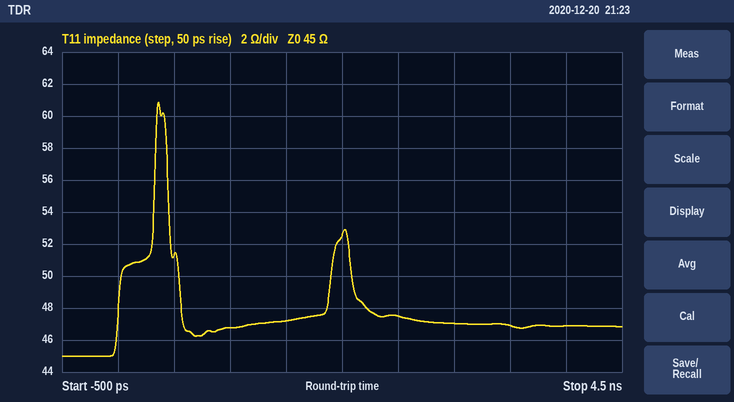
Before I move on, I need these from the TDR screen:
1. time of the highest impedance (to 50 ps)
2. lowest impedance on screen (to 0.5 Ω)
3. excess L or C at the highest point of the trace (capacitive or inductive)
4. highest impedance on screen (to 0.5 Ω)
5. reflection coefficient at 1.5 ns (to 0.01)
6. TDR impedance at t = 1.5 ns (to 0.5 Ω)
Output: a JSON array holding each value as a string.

["350 ps", "45.0 Ω", "inductive", "61.0 Ω", "+0.02", "47.0 Ω"]
